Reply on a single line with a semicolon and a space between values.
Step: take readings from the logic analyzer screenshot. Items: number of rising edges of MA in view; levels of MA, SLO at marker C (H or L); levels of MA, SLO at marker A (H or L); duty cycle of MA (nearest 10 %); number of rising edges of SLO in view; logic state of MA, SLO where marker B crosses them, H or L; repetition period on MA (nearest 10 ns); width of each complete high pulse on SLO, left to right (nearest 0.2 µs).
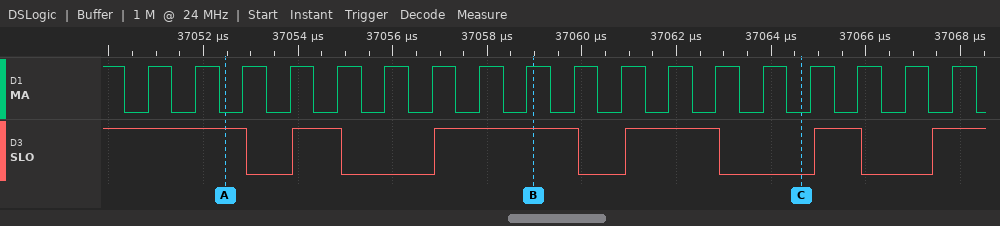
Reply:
18; MA=L, SLO=L; MA=L, SLO=H; 50 %; 5; MA=H, SLO=H; 1000 ns; 1 µs, 3 µs, 2 µs, 1 µs
